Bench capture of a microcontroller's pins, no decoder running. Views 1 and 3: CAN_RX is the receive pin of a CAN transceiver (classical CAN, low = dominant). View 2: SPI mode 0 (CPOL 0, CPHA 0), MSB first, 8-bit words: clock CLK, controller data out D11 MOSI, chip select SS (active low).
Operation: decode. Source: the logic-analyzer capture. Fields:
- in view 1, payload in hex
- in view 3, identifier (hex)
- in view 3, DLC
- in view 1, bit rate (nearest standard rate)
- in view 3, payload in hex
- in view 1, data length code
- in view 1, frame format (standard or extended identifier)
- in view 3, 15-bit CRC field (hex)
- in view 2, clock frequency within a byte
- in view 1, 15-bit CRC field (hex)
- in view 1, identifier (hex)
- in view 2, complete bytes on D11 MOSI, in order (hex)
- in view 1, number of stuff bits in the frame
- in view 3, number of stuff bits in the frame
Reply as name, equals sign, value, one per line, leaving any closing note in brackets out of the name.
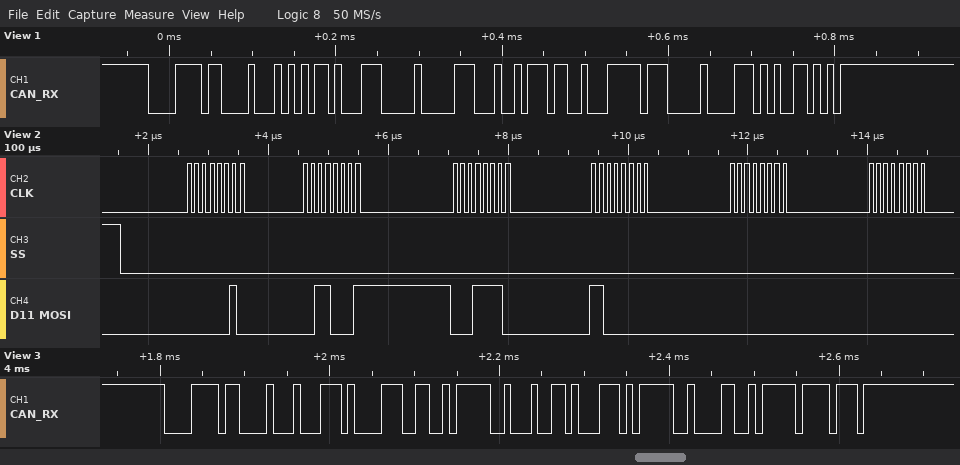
in view 1, payload in hex = AB 47 00 31 2E C8 FF 00
in view 3, identifier = 0x0F6
in view 3, DLC = 8
in view 1, bit rate = 125 kbit/s
in view 3, payload in hex = 8E 87 32 FA 26 8E BE 86
in view 1, data length code = 8
in view 1, frame format = standard
in view 3, 15-bit CRC field = 0x2FFB
in view 2, clock frequency within a byte = 8 MHz
in view 1, 15-bit CRC field = 0x3A9A
in view 1, identifier = 0x0F6
in view 2, complete bytes on D11 MOSI, in order = 02 31 1E C0 00 00
in view 1, number of stuff bits in the frame = 4
in view 3, number of stuff bits in the frame = 3
